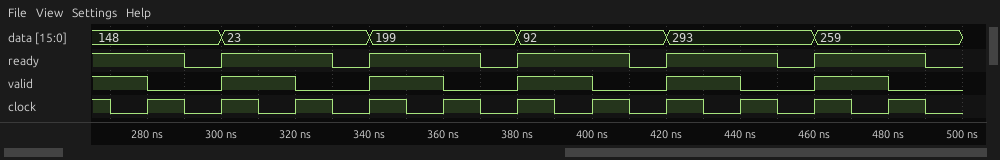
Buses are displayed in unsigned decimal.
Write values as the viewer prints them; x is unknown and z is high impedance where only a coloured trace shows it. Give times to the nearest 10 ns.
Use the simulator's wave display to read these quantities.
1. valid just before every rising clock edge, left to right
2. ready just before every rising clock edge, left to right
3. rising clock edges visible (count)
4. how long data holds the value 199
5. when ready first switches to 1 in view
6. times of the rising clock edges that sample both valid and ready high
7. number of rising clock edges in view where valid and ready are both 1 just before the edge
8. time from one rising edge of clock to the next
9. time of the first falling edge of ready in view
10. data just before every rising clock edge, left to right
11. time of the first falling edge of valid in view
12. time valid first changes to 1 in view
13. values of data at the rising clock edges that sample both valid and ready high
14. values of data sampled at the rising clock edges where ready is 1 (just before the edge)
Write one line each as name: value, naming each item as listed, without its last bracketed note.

valid just before every rising clock edge, left to right: 1 0 1 0 1 0 1 0 1 0 1
ready just before every rising clock edge, left to right: 1 0 1 0 1 0 1 0 1 0 1
rising clock edges visible: 11
how long data holds the value 199: 40 ns
when ready first switches to 1 in view: 300 ns
times of the rising clock edges that sample both valid and ready high: 280 ns, 320 ns, 360 ns, 400 ns, 440 ns, 480 ns
number of rising clock edges in view where valid and ready are both 1 just before the edge: 6
time from one rising edge of clock to the next: 20 ns
time of the first falling edge of ready in view: 290 ns
data just before every rising clock edge, left to right: 148, 148, 23, 23, 199, 199, 92, 92, 293, 293, 259
time of the first falling edge of valid in view: 280 ns
time valid first changes to 1 in view: 300 ns
values of data at the rising clock edges that sample both valid and ready high: 148, 23, 199, 92, 293, 259
values of data sampled at the rising clock edges where ready is 1: 148, 23, 199, 92, 293, 259
